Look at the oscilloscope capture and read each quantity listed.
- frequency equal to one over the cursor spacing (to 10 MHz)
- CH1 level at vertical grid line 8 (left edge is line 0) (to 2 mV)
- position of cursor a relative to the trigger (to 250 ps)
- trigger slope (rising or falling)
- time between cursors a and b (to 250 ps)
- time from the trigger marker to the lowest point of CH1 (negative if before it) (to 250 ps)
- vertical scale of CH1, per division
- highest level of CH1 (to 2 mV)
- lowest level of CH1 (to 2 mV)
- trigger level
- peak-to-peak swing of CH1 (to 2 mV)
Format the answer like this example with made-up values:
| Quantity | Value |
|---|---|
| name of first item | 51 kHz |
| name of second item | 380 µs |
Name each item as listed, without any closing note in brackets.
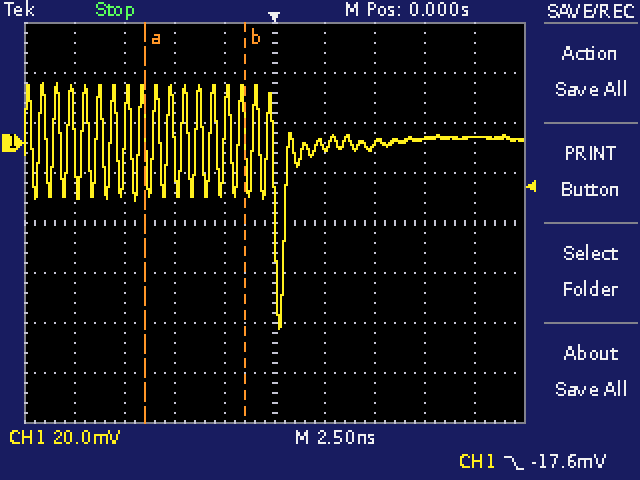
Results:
| Quantity | Value |
|---|---|
| frequency equal to one over the cursor spacing | 200 MHz |
| CH1 level at vertical grid line 8 (left edge is line 0) | 2 mV |
| position of cursor a relative to the trigger | -6.50 ns |
| trigger slope | falling |
| time between cursors a and b | 5.00 ns |
| time from the trigger marker to the lowest point of CH1 (negative if before it) | +250 ps |
| vertical scale of CH1, per division | 20 mV |
| highest level of CH1 | 24 mV |
| lowest level of CH1 | -74 mV |
| trigger level | -17.6 mV |
| peak-to-peak swing of CH1 | 98 mV |
